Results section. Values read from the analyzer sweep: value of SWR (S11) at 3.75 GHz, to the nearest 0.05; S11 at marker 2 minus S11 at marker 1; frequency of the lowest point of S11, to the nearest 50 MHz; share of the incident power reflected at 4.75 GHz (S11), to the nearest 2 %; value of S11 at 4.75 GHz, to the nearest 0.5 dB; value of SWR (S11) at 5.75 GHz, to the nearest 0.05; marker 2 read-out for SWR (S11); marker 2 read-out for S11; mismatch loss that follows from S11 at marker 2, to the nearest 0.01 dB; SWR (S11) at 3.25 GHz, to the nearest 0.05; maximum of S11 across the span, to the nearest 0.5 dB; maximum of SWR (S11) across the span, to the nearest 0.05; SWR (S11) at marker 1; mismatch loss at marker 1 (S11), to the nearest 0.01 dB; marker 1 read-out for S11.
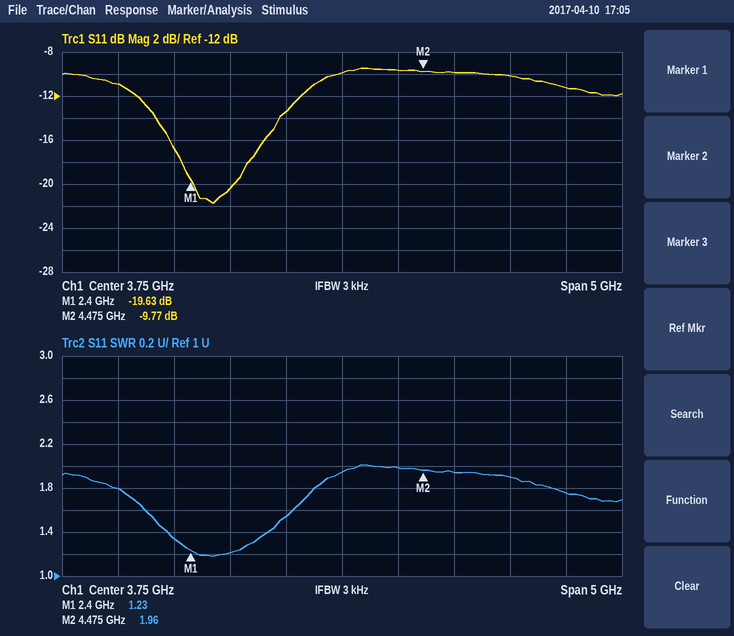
1.95
9.86 dB
2.60 GHz
10 %
-10.0 dB
1.75
1.96
-9.77 dB
0.48 dB
1.55
-9.5 dB
2.00
1.23
0.05 dB
-19.63 dB
